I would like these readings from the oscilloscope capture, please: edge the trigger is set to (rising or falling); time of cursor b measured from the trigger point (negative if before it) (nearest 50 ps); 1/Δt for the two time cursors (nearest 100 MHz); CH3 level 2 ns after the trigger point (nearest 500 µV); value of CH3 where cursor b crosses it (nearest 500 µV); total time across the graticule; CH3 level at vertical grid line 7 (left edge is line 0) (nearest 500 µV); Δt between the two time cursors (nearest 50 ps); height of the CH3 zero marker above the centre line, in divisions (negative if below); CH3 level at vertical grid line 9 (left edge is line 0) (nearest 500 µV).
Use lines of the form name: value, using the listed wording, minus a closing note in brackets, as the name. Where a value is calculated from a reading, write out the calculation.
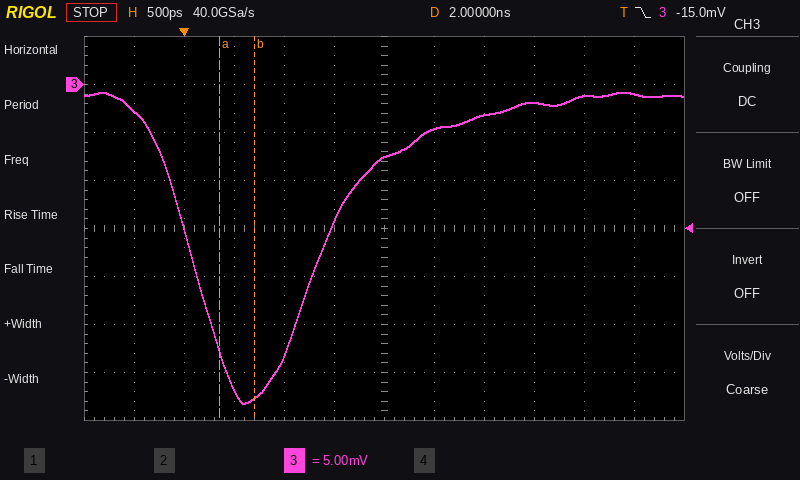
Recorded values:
edge the trigger is set to: falling
time of cursor b measured from the trigger point (negative if before it): +700 ps
1/Δt for the two time cursors: 1 / 350 ps ≈ 2.9 GHz
CH3 level 2 ns after the trigger point: -7.5 mV
value of CH3 where cursor b crosses it: -32.5 mV
total time across the graticule: 6 ns
CH3 level at vertical grid line 7 (left edge is line 0): -4.5 mV
Δt between the two time cursors: 350 ps
height of the CH3 zero marker above the centre line, in divisions: +3.0 div
CH3 level at vertical grid line 9 (left edge is line 0): -2.0 mV
